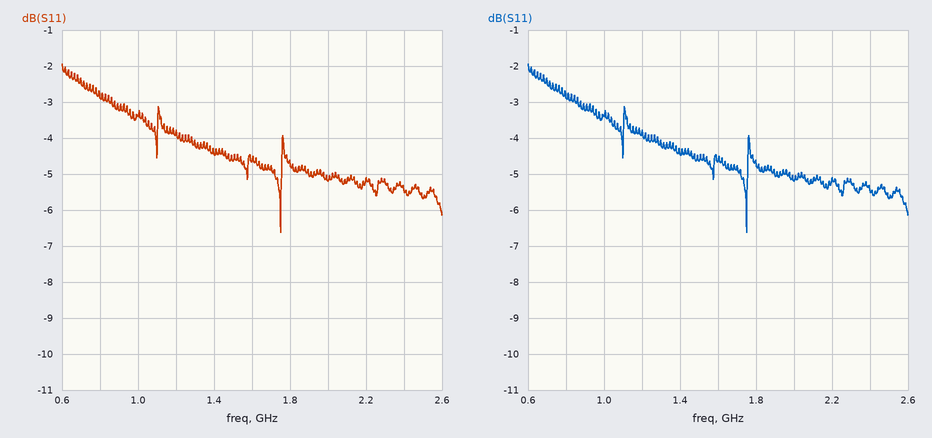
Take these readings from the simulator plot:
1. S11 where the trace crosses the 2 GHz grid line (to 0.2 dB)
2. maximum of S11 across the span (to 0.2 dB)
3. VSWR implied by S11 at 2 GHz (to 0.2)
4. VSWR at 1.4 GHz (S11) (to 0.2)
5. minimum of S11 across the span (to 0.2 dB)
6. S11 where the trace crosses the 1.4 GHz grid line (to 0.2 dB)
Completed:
-5.2 dB
-2.0 dB
3.4
4.0
-6.6 dB
-4.4 dB
